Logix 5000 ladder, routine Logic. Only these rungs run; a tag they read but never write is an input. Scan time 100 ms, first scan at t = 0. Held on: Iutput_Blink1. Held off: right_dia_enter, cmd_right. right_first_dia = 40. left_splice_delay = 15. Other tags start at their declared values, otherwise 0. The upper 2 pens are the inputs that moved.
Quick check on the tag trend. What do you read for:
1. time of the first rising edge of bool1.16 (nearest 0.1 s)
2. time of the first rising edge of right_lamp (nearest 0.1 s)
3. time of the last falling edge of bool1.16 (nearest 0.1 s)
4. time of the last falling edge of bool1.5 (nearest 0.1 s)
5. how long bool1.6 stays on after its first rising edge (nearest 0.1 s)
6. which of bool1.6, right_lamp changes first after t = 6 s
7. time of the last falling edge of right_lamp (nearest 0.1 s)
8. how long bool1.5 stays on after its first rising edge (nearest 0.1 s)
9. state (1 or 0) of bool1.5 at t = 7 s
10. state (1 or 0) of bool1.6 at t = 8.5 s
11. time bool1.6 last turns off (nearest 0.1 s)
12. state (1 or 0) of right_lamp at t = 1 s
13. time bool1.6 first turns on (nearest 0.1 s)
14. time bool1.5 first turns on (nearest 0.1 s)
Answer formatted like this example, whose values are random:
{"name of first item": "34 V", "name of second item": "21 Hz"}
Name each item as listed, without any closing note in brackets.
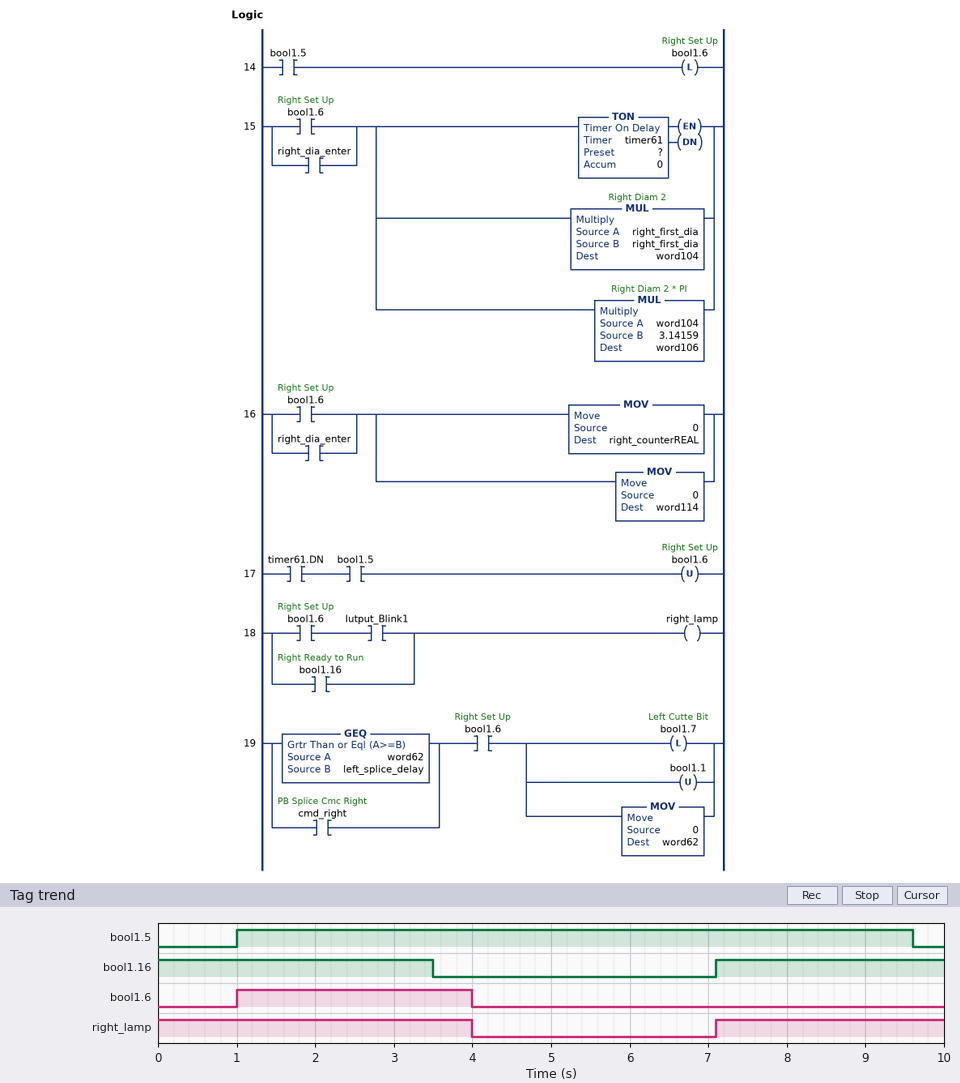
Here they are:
{"time of the first rising edge of bool1.16": "7.1 s", "time of the first rising edge of right_lamp": "7.1 s", "time of the last falling edge of bool1.16": "3.5 s", "time of the last falling edge of bool1.5": "9.6 s", "how long bool1.6 stays on after its first rising edge": "3.0 s", "which of bool1.6, right_lamp changes first after t = 6 s": "right_lamp", "time of the last falling edge of right_lamp": "4.0 s", "how long bool1.5 stays on after its first rising edge": "8.6 s", "state (1 or 0) of bool1.5 at t = 7 s": "1", "state (1 or 0) of bool1.6 at t = 8.5 s": "0", "time bool1.6 last turns off": "4.0 s", "state (1 or 0) of right_lamp at t = 1 s": "1", "time bool1.6 first turns on": "1.0 s", "time bool1.5 first turns on": "1.0 s"}
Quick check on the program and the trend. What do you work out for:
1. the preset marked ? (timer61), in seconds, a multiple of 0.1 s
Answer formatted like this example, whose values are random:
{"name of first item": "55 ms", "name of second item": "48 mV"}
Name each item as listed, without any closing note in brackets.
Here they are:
{"the preset marked ? (timer61), in seconds, a multiple of 0.1 s": "3.0 s"}
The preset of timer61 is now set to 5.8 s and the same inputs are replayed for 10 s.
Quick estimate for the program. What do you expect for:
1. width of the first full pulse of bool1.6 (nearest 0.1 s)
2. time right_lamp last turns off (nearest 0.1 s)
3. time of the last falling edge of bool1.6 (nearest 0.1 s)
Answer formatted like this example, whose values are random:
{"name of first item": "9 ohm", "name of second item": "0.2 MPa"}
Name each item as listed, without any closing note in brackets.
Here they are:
{"width of the first full pulse of bool1.6": "5.8 s", "time right_lamp last turns off": "6.8 s", "time of the last falling edge of bool1.6": "6.8 s"}
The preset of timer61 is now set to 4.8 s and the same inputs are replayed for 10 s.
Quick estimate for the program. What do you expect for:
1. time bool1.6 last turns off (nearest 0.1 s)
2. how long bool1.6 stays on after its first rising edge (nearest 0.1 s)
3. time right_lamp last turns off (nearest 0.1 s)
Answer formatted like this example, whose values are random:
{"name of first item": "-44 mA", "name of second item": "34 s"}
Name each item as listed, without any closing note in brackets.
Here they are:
{"time bool1.6 last turns off": "5.8 s", "how long bool1.6 stays on after its first rising edge": "4.8 s", "time right_lamp last turns off": "5.8 s"}
